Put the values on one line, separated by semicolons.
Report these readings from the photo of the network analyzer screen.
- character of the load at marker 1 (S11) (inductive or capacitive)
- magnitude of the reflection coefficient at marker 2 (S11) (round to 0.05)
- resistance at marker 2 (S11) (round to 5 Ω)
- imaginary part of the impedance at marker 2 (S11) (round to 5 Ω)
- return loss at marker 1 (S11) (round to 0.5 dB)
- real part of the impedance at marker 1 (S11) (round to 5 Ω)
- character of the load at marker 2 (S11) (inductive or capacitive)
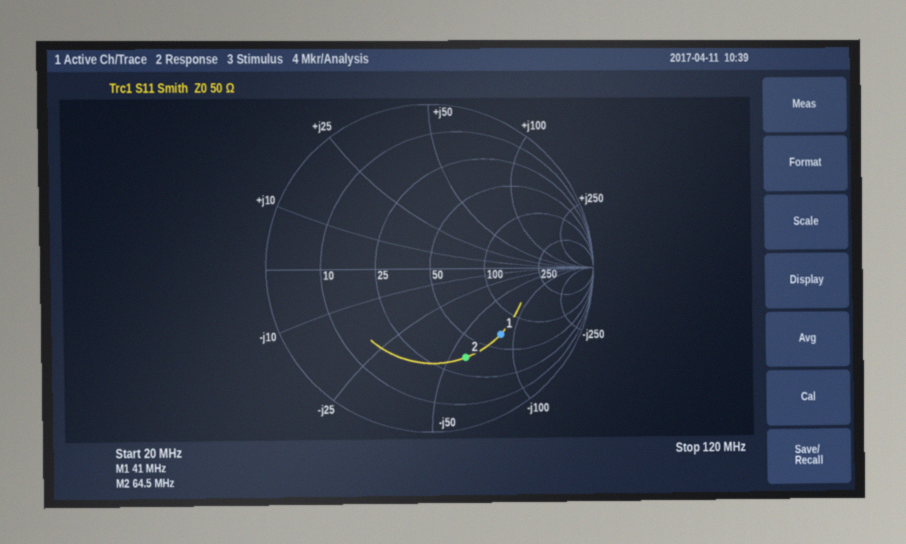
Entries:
capacitive; 0.60; 35 Ω; -60 Ω; 4.5 dB; 65 Ω; capacitive
